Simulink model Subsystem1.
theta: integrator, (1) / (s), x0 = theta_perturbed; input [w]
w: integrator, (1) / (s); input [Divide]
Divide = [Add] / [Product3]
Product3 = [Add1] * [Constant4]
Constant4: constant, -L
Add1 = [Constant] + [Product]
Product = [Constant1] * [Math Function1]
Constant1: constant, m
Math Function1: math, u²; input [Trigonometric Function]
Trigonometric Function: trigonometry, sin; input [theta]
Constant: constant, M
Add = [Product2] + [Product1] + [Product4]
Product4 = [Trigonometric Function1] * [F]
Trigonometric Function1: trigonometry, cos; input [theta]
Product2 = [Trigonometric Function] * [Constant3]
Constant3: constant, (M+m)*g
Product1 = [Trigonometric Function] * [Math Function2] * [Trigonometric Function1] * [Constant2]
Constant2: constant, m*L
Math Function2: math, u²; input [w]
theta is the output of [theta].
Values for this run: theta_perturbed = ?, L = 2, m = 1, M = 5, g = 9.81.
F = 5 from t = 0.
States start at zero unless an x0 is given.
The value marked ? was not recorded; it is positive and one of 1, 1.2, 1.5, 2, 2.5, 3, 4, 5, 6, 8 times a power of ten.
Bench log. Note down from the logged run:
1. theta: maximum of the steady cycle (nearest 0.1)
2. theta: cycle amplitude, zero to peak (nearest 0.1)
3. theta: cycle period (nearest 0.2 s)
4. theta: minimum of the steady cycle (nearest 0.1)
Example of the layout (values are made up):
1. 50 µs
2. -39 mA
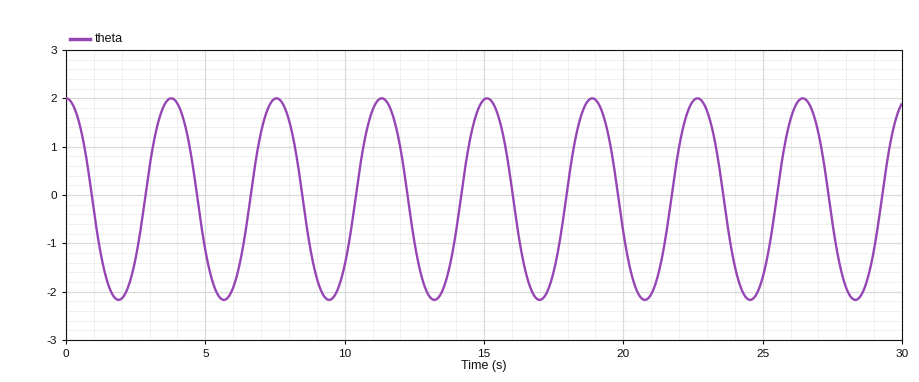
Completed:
1. 2.0
2. 2.1
3. 3.8 s
4. -2.2
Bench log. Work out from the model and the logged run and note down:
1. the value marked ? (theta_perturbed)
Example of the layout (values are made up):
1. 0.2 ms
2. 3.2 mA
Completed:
1. 2
